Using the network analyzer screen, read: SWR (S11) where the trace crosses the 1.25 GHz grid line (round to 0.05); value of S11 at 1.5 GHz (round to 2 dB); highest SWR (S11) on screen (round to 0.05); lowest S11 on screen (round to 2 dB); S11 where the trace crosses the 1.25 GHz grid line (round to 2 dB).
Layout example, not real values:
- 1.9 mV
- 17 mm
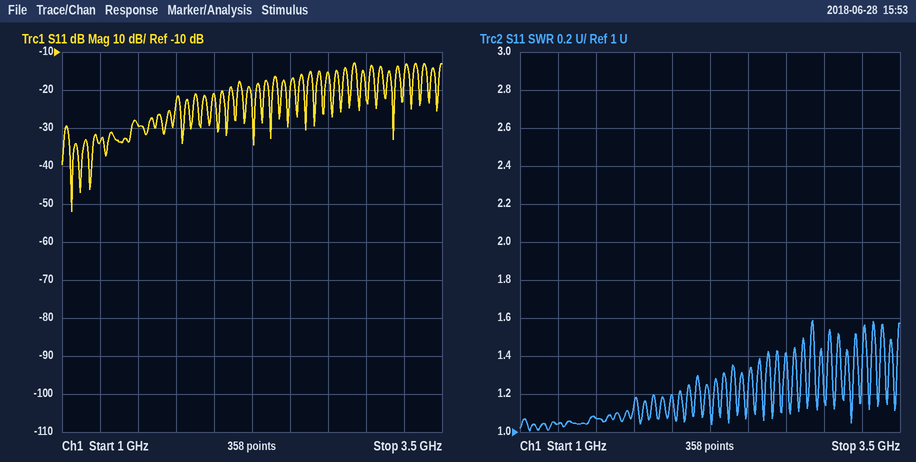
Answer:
- 1.05
- -30 dB
- 1.60
- -52 dB
- -34 dB
